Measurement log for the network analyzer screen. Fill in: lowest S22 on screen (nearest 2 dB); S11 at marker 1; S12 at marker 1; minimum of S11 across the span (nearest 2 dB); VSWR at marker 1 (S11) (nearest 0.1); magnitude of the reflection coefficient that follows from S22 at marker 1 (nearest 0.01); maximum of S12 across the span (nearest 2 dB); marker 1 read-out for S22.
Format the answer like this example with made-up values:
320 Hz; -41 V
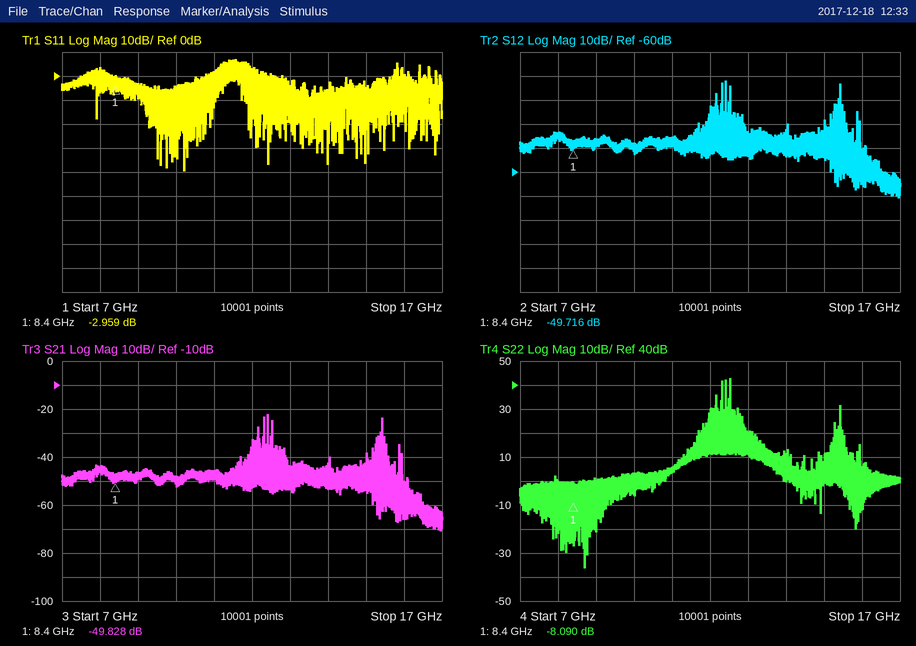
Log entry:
-36 dB; -2.959 dB; -49.716 dB; -40 dB; 5.9; 0.39; -22 dB; -8.090 dB
